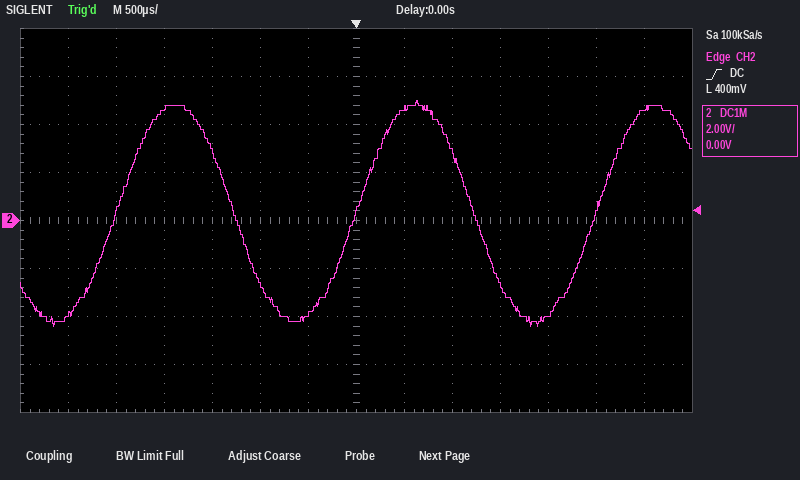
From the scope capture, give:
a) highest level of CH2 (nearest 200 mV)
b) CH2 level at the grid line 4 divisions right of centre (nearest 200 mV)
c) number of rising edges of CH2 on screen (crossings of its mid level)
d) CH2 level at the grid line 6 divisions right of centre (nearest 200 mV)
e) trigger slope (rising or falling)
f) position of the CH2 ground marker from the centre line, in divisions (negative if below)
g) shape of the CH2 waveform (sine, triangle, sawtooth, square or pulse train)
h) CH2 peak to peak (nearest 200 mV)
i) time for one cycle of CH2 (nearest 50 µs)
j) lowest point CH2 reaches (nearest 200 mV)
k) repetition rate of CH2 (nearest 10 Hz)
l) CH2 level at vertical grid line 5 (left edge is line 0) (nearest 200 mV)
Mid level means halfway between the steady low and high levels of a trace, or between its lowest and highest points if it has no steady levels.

5.0 V
-4.0 V
3
4.6 V
rising
0.0 div
sine
9.4 V
2.50 ms
-4.4 V
400 Hz
-2.6 V
